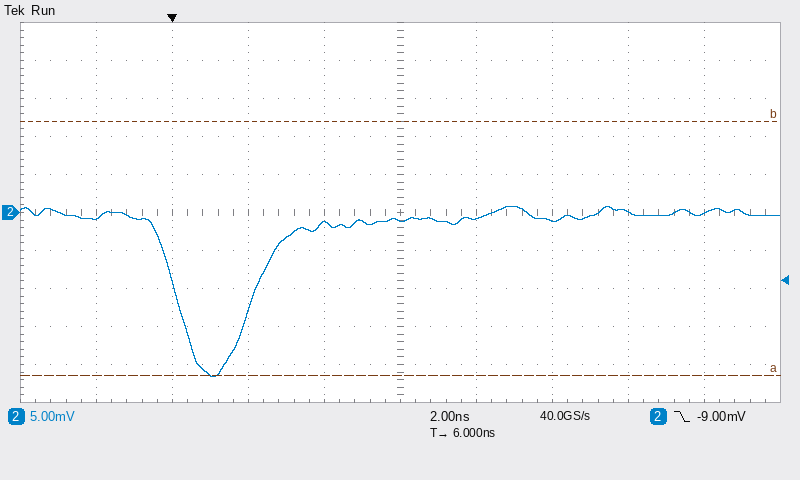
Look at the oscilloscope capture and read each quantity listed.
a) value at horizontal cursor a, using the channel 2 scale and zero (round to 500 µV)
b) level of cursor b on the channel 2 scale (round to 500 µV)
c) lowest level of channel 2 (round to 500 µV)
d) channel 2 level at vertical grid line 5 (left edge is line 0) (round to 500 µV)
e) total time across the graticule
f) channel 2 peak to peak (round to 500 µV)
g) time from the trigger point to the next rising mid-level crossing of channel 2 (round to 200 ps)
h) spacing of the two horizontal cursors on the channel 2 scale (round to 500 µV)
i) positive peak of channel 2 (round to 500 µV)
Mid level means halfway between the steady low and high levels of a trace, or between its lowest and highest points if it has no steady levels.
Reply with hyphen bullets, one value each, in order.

- -21.5 mV
- 12.0 mV
- -21.5 mV
- -1.0 mV
- 20 ns
- 22.5 mV
- 2.2 ns
- 33.5 mV
- 1.0 mV
